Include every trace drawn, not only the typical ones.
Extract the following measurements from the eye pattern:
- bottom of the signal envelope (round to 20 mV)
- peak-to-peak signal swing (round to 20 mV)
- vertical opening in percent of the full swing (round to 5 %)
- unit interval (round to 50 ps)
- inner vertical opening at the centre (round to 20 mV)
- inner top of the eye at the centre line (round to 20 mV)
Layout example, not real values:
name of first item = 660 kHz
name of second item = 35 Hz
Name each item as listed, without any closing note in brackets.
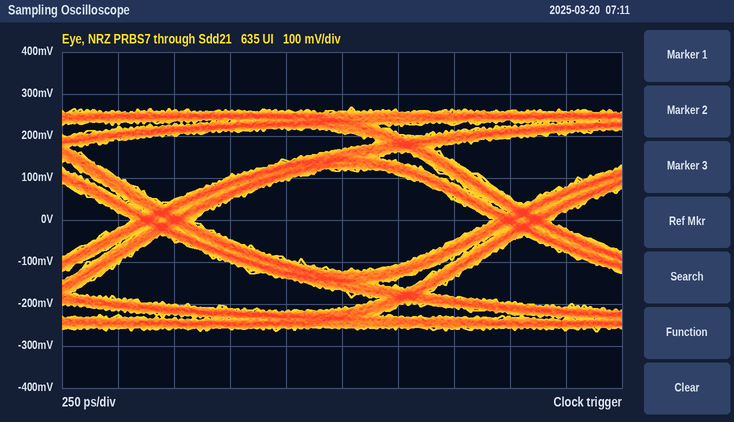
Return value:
bottom of the signal envelope = -260 mV
peak-to-peak signal swing = 540 mV
vertical opening in percent of the full swing = 45 %
unit interval = 1.60 ns
inner vertical opening at the centre = 240 mV
inner top of the eye at the centre line = 120 mV
